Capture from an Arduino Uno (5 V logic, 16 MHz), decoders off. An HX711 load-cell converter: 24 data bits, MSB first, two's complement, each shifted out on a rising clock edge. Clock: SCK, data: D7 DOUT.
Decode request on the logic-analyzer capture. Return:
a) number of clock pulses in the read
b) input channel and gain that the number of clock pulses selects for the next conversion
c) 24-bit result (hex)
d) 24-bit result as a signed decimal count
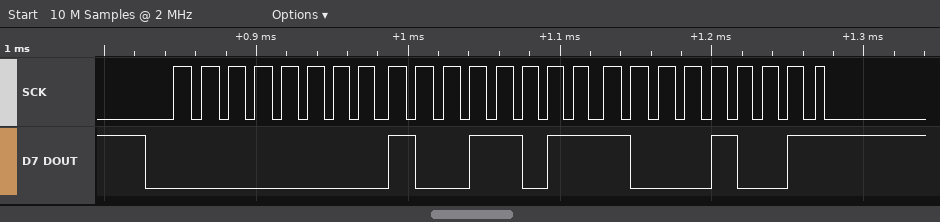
25
channel A, gain 128
0x009B89
39817
